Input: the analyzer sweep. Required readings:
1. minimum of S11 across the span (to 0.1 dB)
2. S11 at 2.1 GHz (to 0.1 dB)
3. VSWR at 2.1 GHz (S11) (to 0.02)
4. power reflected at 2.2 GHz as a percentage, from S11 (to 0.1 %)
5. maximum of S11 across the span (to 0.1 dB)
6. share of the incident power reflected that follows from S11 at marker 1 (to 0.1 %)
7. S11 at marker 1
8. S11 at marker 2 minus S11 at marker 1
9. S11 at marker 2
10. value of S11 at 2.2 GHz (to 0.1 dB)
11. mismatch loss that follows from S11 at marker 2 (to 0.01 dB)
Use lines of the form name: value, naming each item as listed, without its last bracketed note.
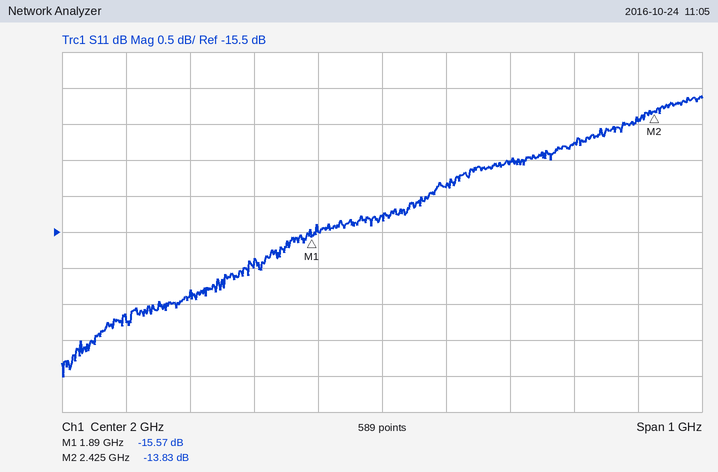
minimum of S11 across the span: -17.5 dB
S11 at 2.1 GHz: -14.9 dB
VSWR at 2.1 GHz (S11): 1.44
power reflected at 2.2 GHz as a percentage, from S11: 3.5 %
maximum of S11 across the span: -13.6 dB
share of the incident power reflected that follows from S11 at marker 1: 2.8 %
S11 at marker 1: -15.57 dB
S11 at marker 2 minus S11 at marker 1: 1.74 dB
S11 at marker 2: -13.83 dB
value of S11 at 2.2 GHz: -14.5 dB
mismatch loss that follows from S11 at marker 2: 0.18 dB
